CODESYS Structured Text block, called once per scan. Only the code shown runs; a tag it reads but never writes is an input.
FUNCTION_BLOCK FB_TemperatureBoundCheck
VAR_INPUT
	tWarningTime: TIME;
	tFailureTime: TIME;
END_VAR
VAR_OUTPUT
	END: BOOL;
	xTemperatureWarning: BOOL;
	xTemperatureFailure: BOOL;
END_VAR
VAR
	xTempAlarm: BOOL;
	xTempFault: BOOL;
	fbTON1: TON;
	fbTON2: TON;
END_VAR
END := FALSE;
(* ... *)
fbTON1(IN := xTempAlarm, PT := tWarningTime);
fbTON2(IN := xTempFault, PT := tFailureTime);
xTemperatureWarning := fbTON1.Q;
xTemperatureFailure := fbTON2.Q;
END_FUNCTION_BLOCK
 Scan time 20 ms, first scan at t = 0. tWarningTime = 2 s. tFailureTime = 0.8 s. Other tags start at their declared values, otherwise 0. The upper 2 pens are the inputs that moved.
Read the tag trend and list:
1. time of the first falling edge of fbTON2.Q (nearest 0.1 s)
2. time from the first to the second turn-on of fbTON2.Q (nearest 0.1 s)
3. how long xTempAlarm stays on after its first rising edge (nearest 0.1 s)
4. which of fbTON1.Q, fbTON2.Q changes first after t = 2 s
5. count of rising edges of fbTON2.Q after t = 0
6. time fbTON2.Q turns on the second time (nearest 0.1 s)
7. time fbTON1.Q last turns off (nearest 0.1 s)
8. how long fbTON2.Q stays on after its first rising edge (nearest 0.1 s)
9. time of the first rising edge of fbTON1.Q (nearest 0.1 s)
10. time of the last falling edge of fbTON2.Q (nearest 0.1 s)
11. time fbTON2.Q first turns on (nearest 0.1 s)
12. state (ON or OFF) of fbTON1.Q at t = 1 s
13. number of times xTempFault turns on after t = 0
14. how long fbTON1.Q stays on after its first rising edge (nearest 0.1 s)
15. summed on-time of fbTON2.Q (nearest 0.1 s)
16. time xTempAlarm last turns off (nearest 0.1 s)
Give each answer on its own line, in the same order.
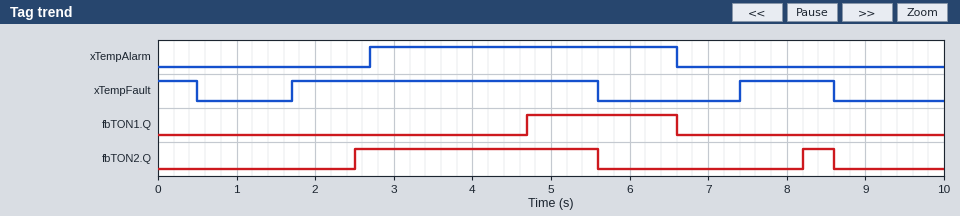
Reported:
5.6 s
5.7 s
3.9 s
fbTON2.Q
2
8.2 s
6.6 s
3.1 s
4.7 s
8.6 s
2.5 s
OFF
2
1.9 s
3.5 s
6.6 s
